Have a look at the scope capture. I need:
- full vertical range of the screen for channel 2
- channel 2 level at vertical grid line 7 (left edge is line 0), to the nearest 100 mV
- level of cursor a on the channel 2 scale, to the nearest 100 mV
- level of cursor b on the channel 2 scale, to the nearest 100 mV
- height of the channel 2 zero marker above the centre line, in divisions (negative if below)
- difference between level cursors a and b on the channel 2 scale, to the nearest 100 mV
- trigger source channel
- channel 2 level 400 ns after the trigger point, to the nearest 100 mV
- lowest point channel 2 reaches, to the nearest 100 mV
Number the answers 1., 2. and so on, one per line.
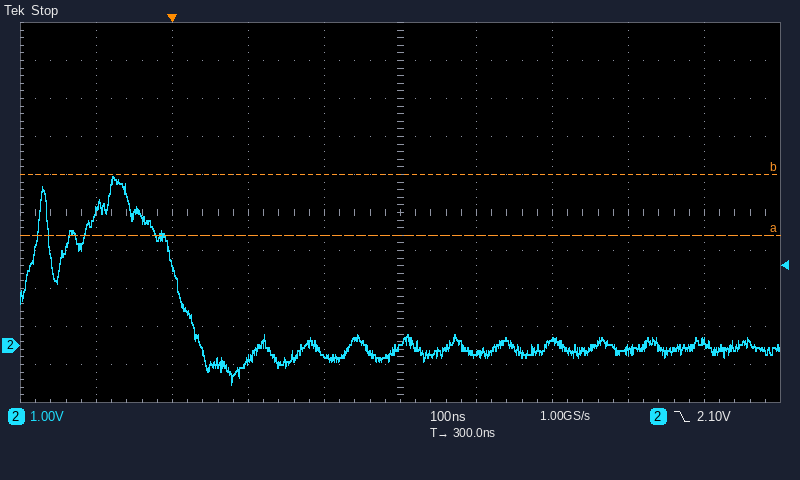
1. 10 V
2. 100 mV
3. 2.9 V
4. 4.5 V
5. -3.5 div
6. 1.6 V
7. channel 2
8. -200 mV
9. -1.0 V
